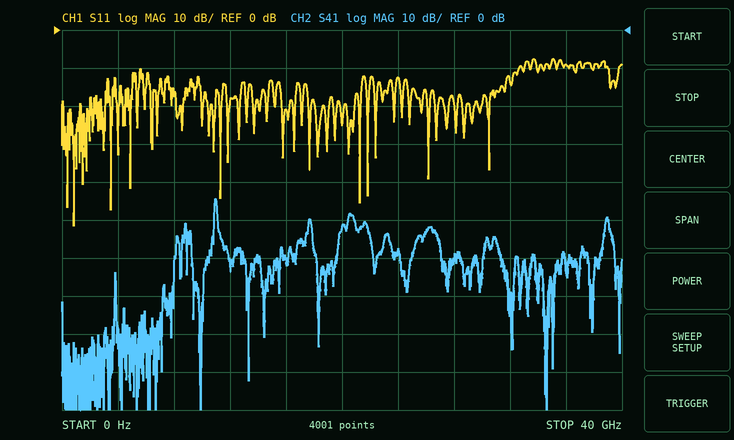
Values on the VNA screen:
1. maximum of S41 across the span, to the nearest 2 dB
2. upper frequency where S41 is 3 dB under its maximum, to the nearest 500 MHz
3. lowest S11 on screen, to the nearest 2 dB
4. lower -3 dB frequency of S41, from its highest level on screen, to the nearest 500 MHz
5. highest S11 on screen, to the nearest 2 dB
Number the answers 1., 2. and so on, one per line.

1. -44 dB
2. 11.0 GHz
3. -52 dB
4. 11.0 GHz
5. -8 dB
